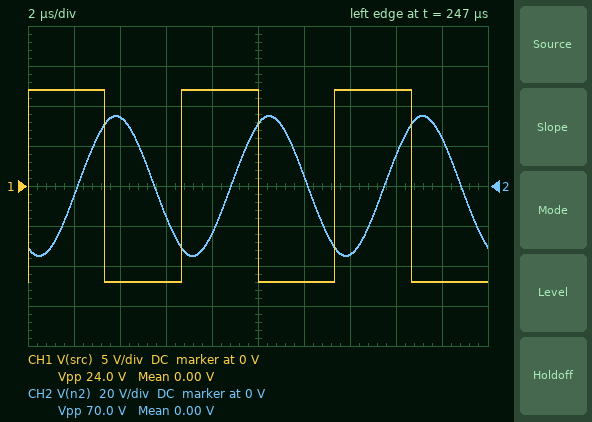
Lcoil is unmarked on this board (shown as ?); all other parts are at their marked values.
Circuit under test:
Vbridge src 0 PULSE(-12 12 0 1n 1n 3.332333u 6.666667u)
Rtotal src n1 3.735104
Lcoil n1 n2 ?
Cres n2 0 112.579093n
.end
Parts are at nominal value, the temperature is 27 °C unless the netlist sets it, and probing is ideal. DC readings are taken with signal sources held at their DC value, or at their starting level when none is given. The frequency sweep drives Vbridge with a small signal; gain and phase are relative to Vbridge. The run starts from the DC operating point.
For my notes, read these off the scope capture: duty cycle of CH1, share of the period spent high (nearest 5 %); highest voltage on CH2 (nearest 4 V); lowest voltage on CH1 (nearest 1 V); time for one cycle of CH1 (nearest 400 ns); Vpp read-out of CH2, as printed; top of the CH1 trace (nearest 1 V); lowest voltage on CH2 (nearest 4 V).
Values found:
50 %
36 V
-12 V
6.8 µs
70.0 V
12 V
-36 V
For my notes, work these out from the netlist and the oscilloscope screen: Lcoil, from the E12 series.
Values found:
12 µH
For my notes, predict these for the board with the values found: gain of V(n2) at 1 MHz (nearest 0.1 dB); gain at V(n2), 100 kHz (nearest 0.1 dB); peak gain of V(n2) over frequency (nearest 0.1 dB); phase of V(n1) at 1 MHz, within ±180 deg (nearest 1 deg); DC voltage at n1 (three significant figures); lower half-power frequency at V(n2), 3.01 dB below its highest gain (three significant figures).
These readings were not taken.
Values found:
-34.4 dB
5.4 dB
9.0 dB
3 deg
-12.0 V
104 kHz
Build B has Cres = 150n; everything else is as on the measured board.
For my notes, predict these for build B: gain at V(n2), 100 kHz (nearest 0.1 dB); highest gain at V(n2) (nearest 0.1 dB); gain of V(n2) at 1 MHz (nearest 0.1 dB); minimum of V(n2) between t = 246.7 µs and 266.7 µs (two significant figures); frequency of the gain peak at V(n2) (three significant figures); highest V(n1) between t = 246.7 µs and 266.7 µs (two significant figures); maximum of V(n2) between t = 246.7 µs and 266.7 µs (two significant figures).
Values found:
6.8 dB
7.8 dB
-36.9 dB
-19 V
113 kHz
21 V
19 V
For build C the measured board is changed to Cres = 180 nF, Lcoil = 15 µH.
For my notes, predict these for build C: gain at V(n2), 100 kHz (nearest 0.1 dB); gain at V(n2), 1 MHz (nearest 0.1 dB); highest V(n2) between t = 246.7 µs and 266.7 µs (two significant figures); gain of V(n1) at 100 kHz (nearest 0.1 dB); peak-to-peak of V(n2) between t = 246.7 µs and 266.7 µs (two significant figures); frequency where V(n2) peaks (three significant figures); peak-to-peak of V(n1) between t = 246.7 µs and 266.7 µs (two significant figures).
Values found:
7.4 dB
-40.5 dB
9.9 V
-16.2 dB
20 V
92.7 kHz
37 V
